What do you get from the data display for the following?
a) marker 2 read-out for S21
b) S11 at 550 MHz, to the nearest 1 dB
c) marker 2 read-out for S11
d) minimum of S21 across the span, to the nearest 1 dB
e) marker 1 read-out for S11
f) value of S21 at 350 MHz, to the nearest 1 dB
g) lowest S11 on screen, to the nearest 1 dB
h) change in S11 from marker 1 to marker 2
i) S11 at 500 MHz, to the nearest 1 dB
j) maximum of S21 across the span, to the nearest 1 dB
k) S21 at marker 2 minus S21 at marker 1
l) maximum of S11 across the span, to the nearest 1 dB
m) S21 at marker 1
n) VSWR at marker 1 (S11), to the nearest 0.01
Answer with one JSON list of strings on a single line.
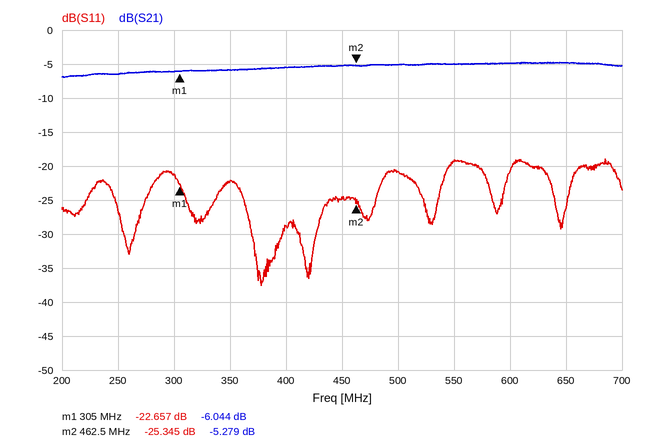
["-5.279 dB", "-19 dB", "-25.345 dB", "-7 dB", "-22.657 dB", "-6 dB", "-38 dB", "-2.688 dB", "-21 dB", "-5 dB", "0.765 dB", "-19 dB", "-6.044 dB", "1.16"]
